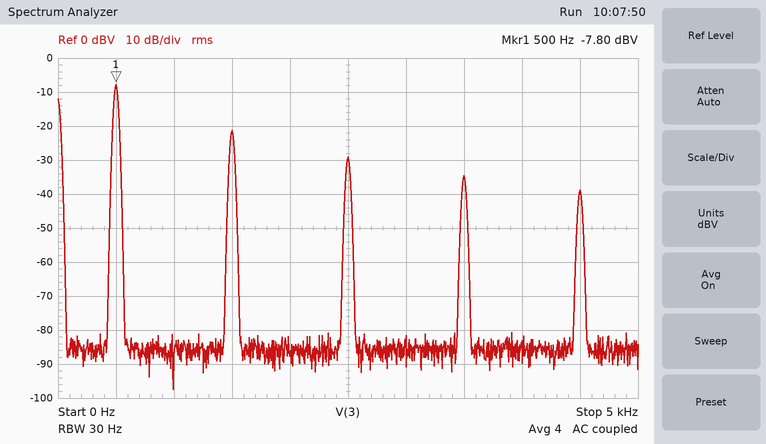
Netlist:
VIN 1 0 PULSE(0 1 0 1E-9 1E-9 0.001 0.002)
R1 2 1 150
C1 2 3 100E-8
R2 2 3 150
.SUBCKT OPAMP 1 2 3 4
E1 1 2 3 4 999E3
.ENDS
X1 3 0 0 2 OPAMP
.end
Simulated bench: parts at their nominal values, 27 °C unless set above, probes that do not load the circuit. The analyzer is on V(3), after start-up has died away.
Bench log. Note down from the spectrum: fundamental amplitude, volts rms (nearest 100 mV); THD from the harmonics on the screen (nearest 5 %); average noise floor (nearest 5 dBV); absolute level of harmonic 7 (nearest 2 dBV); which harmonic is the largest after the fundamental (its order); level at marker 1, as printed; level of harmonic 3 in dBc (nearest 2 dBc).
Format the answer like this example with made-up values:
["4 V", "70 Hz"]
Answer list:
["400 mV", "25 %", "-85 dBV", "-34 dBV", "3", "-7.80 dBV", "-14 dBc"]
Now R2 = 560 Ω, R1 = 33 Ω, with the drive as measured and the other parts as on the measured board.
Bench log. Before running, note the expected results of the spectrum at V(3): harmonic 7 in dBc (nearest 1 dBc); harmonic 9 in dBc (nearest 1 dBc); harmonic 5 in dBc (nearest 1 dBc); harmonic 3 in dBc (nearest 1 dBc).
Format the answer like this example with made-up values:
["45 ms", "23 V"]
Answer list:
["-33 dBc", "-37 dBc", "-27 dBc", "-18 dBc"]
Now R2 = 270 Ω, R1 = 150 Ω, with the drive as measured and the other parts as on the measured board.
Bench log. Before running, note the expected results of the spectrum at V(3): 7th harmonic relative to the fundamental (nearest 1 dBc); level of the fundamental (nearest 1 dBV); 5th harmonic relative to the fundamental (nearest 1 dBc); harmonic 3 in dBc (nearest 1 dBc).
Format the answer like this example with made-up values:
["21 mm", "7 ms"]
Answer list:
["-30 dBc", "-4 dBV", "-24 dBc", "-16 dBc"]
